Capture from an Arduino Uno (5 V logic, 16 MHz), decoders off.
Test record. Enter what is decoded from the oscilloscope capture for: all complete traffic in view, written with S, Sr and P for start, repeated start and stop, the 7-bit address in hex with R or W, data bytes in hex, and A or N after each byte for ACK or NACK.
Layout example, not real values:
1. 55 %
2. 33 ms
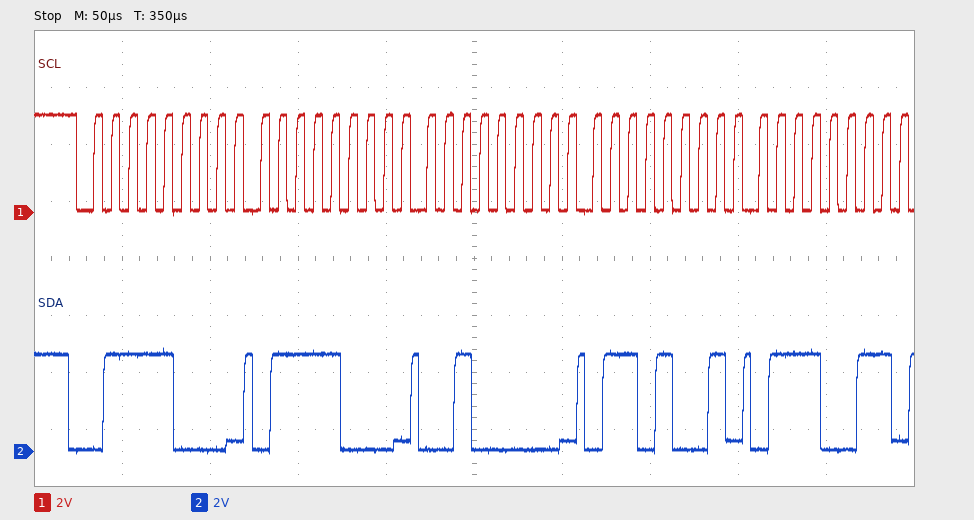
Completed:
1. S 3CW A 78 A 20 A 69 A 73 A
